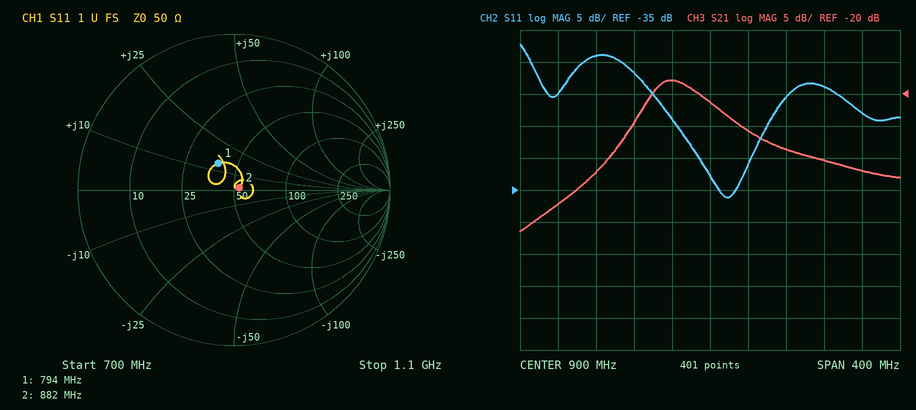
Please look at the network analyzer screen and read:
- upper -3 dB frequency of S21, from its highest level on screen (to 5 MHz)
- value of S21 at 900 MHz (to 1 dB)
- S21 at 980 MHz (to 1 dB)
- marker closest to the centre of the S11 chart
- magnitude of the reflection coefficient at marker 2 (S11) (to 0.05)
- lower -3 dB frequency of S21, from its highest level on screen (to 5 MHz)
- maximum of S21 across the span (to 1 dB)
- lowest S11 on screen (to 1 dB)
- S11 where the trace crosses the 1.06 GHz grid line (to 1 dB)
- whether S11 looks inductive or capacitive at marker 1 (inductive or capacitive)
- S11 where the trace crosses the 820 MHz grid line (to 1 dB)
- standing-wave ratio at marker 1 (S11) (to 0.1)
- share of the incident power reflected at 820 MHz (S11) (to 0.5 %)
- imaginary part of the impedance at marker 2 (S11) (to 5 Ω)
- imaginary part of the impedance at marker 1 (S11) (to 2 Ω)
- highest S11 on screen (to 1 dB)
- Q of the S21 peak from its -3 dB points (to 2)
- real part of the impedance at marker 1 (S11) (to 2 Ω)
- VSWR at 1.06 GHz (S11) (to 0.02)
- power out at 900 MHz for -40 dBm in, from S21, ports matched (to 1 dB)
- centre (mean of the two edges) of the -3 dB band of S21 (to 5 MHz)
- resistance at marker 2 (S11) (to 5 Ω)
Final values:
895 MHz
-21 dB
-29 dB
marker 2
0.05
835 MHz
-18 dB
-36 dB
-23 dB
inductive
-17 dB
1.5
2.0 %
0 Ω
+14 Ω
-12 dB
14
38 Ω
1.16
-61 dBm
865 MHz
55 Ω
